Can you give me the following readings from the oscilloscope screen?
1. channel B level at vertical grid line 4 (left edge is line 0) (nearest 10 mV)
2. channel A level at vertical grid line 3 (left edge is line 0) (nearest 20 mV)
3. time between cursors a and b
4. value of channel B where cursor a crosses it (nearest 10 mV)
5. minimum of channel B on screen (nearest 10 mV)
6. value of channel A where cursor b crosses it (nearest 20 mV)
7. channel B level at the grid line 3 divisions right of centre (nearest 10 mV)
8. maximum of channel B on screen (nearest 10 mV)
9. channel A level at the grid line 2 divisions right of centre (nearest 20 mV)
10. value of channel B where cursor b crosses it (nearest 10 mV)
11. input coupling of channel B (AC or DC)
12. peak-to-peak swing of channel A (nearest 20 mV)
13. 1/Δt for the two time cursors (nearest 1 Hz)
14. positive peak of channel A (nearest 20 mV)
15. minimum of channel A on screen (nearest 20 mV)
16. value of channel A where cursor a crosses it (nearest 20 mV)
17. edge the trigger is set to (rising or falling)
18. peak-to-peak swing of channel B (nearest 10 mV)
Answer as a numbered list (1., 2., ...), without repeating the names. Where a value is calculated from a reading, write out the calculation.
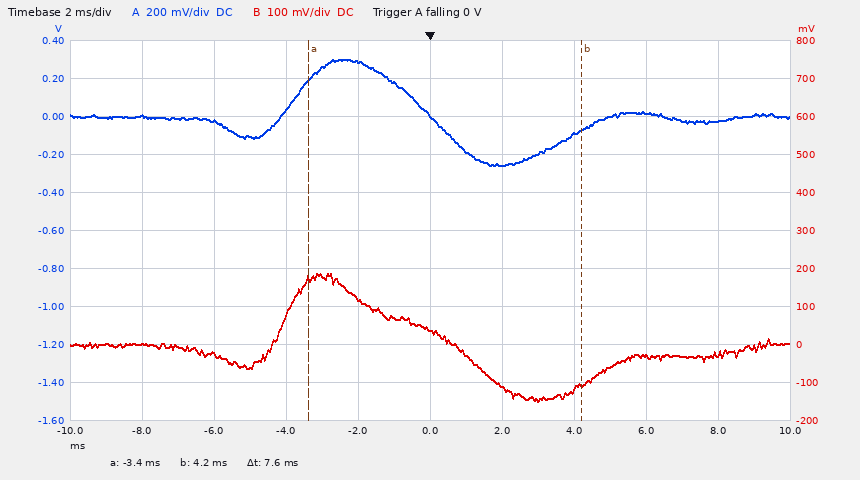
1. 120 mV
2. 40 mV
3. 7.6 ms
4. 170 mV
5. -150 mV
6. -80 mV
7. -30 mV
8. 190 mV
9. -100 mV
10. -110 mV
11. DC
12. 300 mV − (-260 mV) = 560 mV
13. 1 / 7.6 ms ≈ 132 Hz
14. 300 mV
15. -260 mV
16. 200 mV
17. falling
18. 190 mV − (-150 mV) = 340 mV
